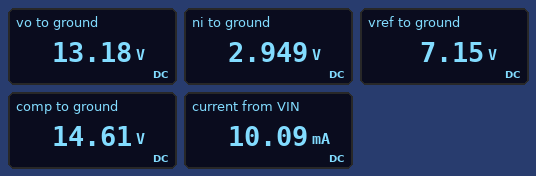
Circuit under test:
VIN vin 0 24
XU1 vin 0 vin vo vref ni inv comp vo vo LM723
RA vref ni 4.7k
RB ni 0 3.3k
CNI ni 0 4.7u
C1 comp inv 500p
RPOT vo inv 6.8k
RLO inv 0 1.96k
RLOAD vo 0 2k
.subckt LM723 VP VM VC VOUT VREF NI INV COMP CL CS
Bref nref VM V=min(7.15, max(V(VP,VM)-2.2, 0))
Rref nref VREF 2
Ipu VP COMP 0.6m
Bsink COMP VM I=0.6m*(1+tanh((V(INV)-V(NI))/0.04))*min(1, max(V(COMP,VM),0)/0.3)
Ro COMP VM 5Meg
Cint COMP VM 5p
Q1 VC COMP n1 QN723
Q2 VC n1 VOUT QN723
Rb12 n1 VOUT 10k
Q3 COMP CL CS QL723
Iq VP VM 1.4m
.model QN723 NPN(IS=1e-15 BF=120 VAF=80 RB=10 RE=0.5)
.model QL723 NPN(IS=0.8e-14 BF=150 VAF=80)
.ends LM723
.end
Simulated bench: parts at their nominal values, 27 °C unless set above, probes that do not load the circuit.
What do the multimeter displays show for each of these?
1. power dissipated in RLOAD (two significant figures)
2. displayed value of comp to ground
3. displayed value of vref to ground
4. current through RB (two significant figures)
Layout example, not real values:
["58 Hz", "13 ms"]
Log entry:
["87 mW", "14.61 V", "7.15 V", "890 µA"]
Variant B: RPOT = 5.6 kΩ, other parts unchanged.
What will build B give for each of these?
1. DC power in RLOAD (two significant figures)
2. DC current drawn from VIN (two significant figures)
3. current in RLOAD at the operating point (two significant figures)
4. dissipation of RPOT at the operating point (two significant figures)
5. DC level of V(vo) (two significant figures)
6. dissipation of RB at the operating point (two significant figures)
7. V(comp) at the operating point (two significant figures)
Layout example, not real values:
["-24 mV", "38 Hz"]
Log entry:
["65 mW", "9.2 mA", "5.7 mA", "13 mW", "11 V", "2.6 mW", "13 V"]
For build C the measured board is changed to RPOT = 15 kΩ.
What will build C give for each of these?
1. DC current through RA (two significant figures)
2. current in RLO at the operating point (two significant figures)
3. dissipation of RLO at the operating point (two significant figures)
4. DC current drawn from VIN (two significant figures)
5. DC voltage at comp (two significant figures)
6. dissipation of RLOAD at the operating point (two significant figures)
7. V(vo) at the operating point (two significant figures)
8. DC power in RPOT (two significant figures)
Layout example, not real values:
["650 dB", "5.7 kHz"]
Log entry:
["890 µA", "1.4 mA", "3.7 mW", "14 mA", "25 V", "270 mW", "23 V", "28 mW"]
